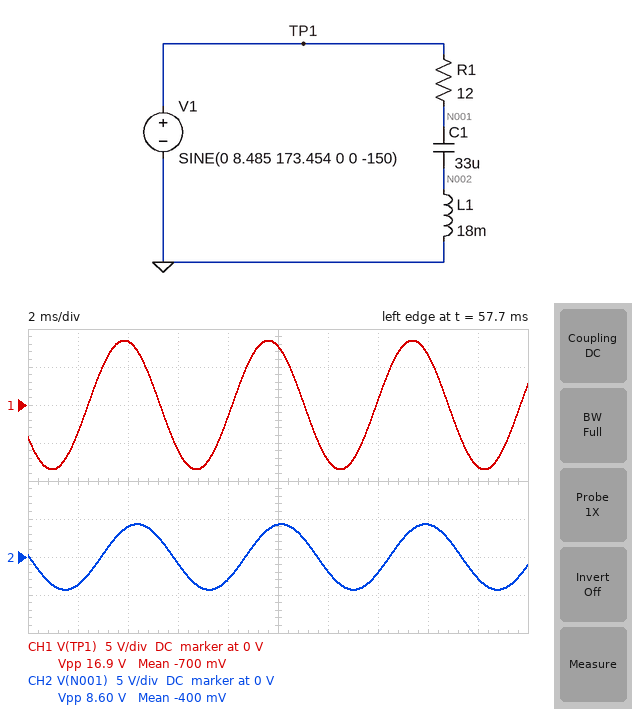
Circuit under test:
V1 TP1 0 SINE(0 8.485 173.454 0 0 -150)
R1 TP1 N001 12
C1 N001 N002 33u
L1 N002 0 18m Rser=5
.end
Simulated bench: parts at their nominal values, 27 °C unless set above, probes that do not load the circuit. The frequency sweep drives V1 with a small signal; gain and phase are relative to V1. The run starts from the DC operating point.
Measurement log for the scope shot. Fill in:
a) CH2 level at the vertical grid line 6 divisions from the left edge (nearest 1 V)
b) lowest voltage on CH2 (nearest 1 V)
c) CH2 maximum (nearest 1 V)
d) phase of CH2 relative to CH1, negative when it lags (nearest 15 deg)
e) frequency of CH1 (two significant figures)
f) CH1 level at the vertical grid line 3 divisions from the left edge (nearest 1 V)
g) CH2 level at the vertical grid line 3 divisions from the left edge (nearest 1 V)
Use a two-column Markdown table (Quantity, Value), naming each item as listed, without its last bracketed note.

| Quantity | Value |
|---|---|
| CH2 level at the vertical grid line 6 divisions from the left edge | -2 V |
| lowest voltage on CH2 | -4 V |
| CH2 maximum | 4 V |
| phase of CH2 relative to CH1, negative when it lags | -30 deg |
| frequency of CH1 | 170 Hz |
| CH1 level at the vertical grid line 3 divisions from the left edge | -6 V |
| CH2 level at the vertical grid line 3 divisions from the left edge | -1 V |
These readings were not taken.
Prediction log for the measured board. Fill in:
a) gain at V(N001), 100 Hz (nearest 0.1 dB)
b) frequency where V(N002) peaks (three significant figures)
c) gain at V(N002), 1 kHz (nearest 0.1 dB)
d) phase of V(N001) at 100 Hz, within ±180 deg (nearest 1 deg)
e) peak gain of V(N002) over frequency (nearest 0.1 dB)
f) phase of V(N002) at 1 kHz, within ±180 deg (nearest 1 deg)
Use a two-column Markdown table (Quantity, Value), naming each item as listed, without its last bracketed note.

| Quantity | Value |
|---|---|
| gain at V(N001), 100 Hz | -0.8 dB |
| frequency where V(N002) peaks | 239 Hz |
| gain at V(N002), 1 kHz | 0.3 dB |
| phase of V(N001) at 100 Hz, within ±180 deg | -17 deg |
| peak gain of V(N002) over frequency | 3.5 dB |
| phase of V(N002) at 1 kHz, within ±180 deg | 6 deg |
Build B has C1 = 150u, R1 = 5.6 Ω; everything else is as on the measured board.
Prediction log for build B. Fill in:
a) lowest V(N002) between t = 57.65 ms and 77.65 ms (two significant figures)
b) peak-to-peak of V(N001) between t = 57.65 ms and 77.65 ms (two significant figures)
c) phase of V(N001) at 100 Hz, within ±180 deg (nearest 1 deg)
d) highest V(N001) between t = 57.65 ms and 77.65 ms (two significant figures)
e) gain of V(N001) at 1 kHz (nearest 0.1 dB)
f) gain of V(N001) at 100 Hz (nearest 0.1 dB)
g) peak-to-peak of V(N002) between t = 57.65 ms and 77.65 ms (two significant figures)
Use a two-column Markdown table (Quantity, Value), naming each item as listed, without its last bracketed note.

| Quantity | Value |
|---|---|
| lowest V(N002) between t = 57.65 ms and 77.65 ms | -10 V |
| peak-to-peak of V(N001) between t = 57.65 ms and 77.65 ms | 14 V |
| phase of V(N001) at 100 Hz, within ±180 deg | 4 deg |
| highest V(N001) between t = 57.65 ms and 77.65 ms | 7.1 V |
| gain of V(N001) at 1 kHz | 0 dB |
| gain of V(N001) at 100 Hz | -6.5 dB |
| peak-to-peak of V(N002) between t = 57.65 ms and 77.65 ms | 20 V |
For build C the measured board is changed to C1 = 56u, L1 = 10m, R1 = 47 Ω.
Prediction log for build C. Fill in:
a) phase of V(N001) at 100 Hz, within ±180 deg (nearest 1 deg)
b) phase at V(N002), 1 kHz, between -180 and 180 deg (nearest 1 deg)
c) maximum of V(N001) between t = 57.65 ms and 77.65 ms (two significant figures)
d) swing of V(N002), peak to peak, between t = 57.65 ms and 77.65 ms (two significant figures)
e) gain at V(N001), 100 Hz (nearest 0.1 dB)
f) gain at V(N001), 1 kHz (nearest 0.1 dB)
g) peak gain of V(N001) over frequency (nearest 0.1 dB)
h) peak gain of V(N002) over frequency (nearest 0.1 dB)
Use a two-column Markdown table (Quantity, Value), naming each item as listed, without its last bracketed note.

| Quantity | Value |
|---|---|
| phase of V(N001) at 100 Hz, within ±180 deg | -54 deg |
| phase at V(N002), 1 kHz, between -180 and 180 deg | 36 deg |
| maximum of V(N001) between t = 57.65 ms and 77.65 ms | 1.2 V |
| swing of V(N002), peak to peak, between t = 57.65 ms and 77.65 ms | 3.9 V |
| gain at V(N001), 100 Hz | -7.9 dB |
| gain at V(N001), 1 kHz | -2.4 dB |
| peak gain of V(N001) over frequency | 0 dB |
| peak gain of V(N002) over frequency | 0 dB |
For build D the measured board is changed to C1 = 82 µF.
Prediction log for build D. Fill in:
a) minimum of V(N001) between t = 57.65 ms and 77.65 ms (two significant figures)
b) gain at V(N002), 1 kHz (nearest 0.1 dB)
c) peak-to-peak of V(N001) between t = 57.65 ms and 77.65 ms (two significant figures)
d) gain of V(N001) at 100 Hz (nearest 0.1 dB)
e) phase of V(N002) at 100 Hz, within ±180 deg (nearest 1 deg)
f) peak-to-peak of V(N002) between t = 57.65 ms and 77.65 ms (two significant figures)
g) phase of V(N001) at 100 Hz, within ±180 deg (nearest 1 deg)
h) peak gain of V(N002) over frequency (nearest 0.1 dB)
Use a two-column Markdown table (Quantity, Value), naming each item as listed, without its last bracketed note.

| Quantity | Value |
|---|---|
| minimum of V(N001) between t = 57.65 ms and 77.65 ms | -4.4 V |
| gain at V(N002), 1 kHz | 0.1 dB |
| peak-to-peak of V(N001) between t = 57.65 ms and 77.65 ms | 8.8 V |
| gain of V(N001) at 100 Hz | -5.9 dB |
| phase of V(N002) at 100 Hz, within ±180 deg | 92 deg |
| peak-to-peak of V(N002) between t = 57.65 ms and 77.65 ms | 18 V |
| phase of V(N001) at 100 Hz, within ±180 deg | -33 deg |
| peak gain of V(N002) over frequency | 0.7 dB |
